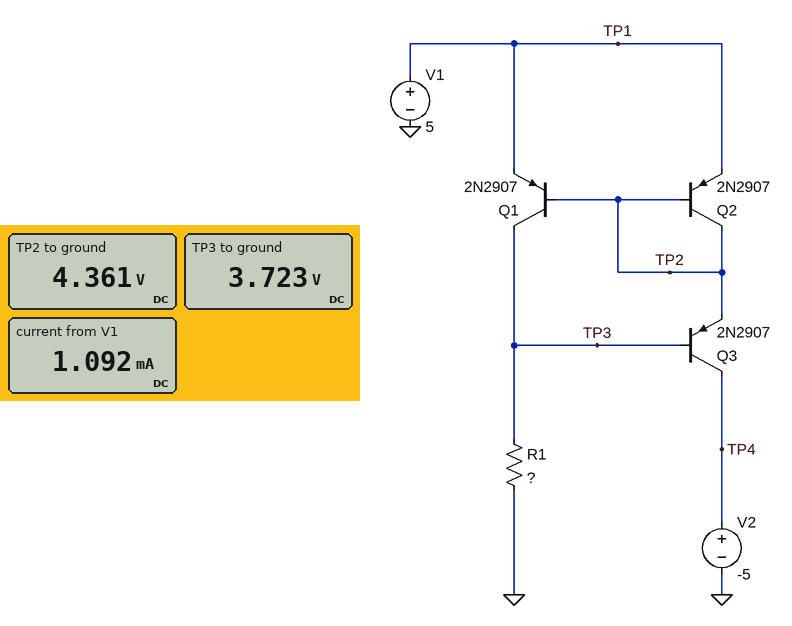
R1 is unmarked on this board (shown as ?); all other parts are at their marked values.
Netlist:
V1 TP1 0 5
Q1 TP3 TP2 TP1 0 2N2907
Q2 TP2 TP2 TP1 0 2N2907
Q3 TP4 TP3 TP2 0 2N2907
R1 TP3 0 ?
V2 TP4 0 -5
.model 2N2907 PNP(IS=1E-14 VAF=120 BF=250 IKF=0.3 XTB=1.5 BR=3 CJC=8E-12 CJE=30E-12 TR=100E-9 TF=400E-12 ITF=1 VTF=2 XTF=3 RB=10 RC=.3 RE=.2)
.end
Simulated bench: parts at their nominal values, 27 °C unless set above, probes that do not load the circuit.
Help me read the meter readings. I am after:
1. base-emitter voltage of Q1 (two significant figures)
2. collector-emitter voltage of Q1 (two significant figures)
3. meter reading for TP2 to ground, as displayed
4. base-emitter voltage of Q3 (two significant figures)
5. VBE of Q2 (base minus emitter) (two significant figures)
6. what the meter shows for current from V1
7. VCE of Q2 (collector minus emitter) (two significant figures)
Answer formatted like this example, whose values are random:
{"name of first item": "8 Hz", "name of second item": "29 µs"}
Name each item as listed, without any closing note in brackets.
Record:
{"base-emitter voltage of Q1": "-640 mV", "collector-emitter voltage of Q1": "-1.3 V", "meter reading for TP2 to ground, as displayed": "4.361 V", "base-emitter voltage of Q3": "-640 mV", "VBE of Q2 (base minus emitter)": "-640 mV", "what the meter shows for current from V1": "1.092 mA", "VCE of Q2 (collector minus emitter)": "-640 mV"}
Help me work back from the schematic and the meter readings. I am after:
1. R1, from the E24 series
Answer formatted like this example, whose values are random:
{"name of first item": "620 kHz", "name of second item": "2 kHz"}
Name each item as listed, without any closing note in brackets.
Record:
{"R1, from the E24 series": "6.8 kΩ"}
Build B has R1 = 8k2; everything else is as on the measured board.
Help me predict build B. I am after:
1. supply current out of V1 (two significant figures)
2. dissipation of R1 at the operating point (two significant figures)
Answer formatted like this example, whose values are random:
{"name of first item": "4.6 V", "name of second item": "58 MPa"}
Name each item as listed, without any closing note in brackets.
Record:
{"supply current out of V1": "910 µA", "dissipation of R1 at the operating point": "1.7 mW"}
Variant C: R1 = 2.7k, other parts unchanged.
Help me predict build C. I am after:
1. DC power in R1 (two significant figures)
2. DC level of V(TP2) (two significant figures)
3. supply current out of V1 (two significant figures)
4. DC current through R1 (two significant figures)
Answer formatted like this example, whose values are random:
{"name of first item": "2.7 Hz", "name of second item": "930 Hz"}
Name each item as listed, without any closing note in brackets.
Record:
{"DC power in R1": "5.0 mW", "DC level of V(TP2)": "4.3 V", "supply current out of V1": "2.7 mA", "DC current through R1": "1.4 mA"}
